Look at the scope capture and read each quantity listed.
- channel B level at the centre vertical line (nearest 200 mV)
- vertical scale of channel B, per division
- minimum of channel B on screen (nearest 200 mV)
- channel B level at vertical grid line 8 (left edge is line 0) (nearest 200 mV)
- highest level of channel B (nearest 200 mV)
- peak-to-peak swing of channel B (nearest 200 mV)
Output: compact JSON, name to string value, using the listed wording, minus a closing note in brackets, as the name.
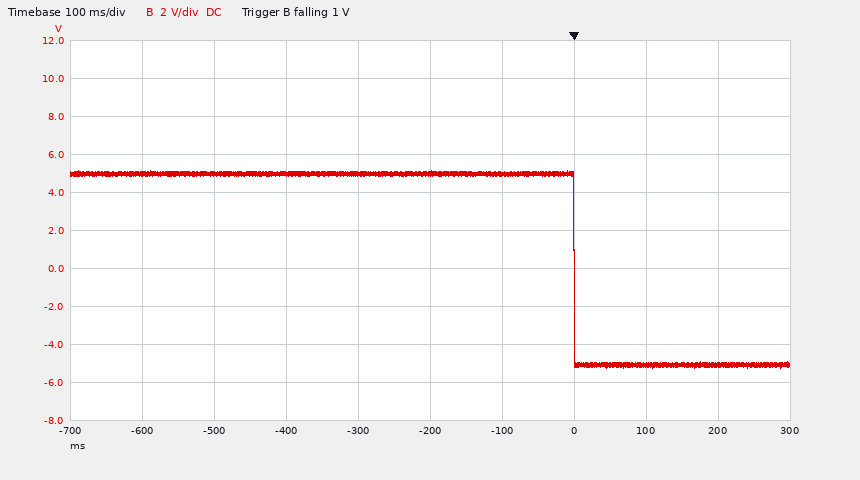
{"channel B level at the centre vertical line": "5.0 V", "vertical scale of channel B, per division": "2 V", "minimum of channel B on screen": "-5.2 V", "channel B level at vertical grid line 8 (left edge is line 0)": "-5.0 V", "highest level of channel B": "5.2 V", "peak-to-peak swing of channel B": "10.4 V"}
